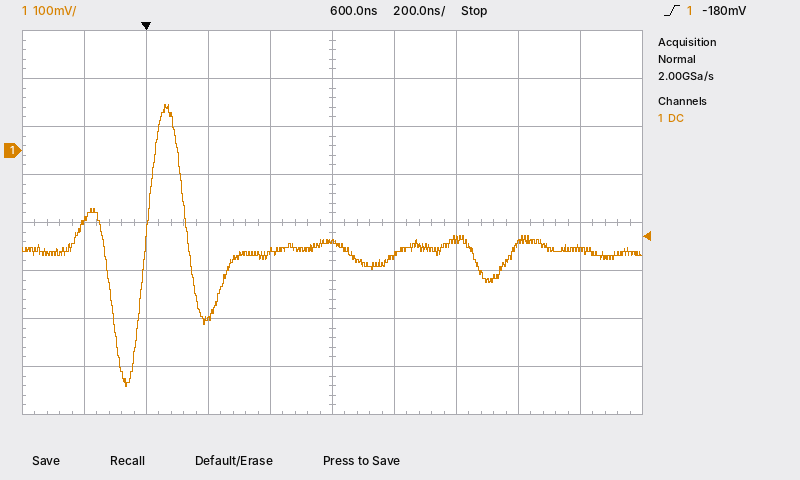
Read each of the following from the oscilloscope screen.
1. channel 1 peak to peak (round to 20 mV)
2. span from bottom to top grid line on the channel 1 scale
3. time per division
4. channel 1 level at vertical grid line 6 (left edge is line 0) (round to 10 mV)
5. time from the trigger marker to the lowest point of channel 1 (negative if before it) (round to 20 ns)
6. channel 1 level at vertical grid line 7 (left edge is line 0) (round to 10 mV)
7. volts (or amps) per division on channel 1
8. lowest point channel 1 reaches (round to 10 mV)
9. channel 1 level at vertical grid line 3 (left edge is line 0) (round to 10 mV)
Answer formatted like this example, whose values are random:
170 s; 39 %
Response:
580 mV; 800 mV; 200 ns; -220 mV; -60 ns; -190 mV; 100 mV; -490 mV; -350 mV
